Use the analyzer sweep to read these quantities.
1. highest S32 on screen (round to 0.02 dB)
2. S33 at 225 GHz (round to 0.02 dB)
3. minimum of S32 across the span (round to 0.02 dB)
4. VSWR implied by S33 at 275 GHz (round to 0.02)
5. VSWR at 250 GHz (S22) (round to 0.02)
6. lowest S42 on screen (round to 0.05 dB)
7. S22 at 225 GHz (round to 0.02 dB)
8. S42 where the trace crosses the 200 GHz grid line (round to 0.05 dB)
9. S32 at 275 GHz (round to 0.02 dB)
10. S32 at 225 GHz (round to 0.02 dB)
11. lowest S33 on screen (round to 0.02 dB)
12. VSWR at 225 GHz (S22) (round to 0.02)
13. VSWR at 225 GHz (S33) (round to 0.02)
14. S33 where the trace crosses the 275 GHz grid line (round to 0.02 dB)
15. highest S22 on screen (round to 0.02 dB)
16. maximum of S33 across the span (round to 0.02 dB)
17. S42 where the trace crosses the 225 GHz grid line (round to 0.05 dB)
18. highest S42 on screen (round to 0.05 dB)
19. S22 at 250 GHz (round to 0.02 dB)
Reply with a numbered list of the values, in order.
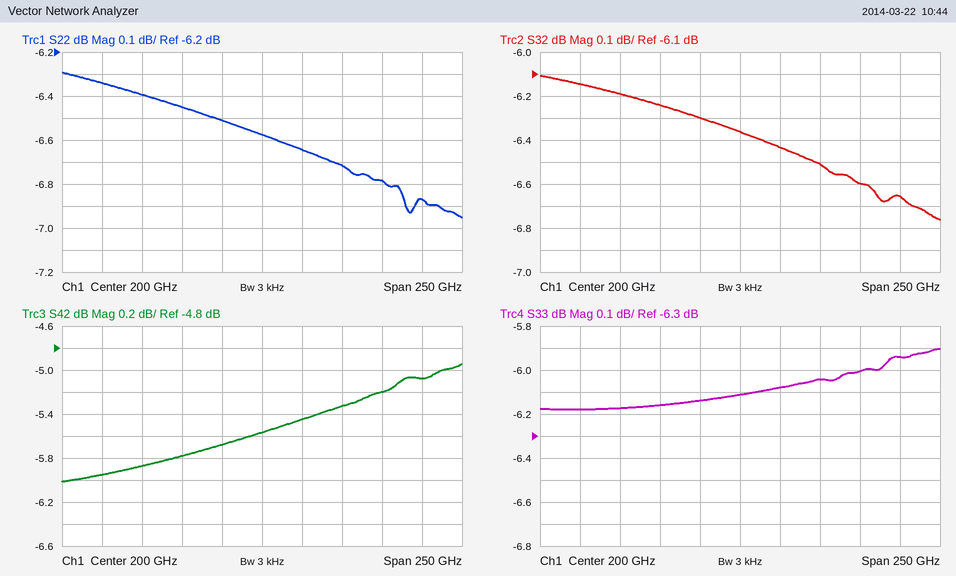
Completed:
1. -6.10 dB
2. -6.08 dB
3. -6.76 dB
4. 3.00
5. 2.72
6. -6.00 dB
7. -6.64 dB
8. -5.55 dB
9. -6.60 dB
10. -6.44 dB
11. -6.18 dB
12. 2.74
13. 2.98
14. -6.00 dB
15. -6.30 dB
16. -5.90 dB
17. -5.45 dB
18. -4.95 dB
19. -6.72 dB
